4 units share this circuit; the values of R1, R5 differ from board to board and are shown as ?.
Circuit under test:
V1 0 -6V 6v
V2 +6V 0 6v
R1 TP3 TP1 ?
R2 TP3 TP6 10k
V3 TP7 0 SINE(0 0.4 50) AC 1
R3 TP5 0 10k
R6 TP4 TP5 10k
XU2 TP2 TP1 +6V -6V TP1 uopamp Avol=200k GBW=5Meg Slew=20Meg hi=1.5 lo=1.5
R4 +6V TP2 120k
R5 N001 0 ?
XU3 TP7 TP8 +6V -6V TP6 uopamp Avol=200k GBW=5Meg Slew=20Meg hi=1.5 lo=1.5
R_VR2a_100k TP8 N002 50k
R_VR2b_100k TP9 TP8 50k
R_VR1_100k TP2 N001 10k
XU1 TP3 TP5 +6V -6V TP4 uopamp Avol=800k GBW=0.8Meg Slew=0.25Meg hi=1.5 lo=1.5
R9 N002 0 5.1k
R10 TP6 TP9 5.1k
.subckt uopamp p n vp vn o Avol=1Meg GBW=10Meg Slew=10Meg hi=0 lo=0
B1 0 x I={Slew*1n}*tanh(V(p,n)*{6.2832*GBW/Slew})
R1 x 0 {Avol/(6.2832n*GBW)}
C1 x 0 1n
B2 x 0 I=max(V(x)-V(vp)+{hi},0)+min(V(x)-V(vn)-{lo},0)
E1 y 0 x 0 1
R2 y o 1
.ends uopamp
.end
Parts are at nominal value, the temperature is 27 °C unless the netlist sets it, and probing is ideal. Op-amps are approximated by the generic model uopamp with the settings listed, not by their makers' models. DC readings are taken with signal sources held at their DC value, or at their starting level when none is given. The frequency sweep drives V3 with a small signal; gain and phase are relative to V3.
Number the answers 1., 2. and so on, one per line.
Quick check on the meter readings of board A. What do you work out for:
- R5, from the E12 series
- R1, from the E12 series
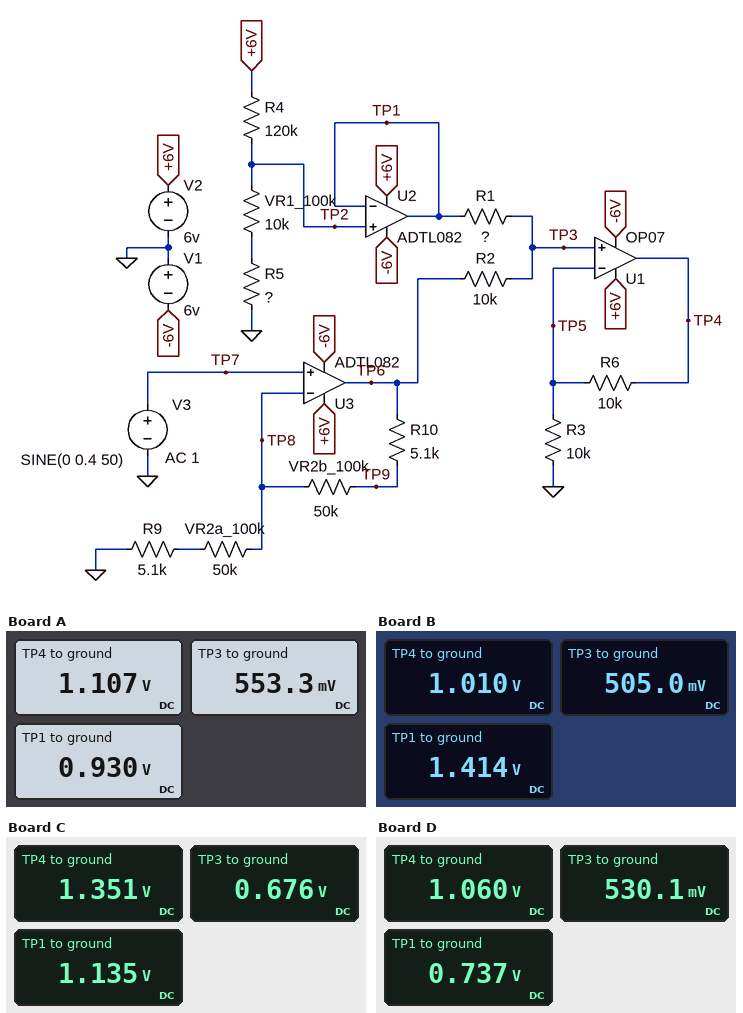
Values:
1. 12 kΩ
2. 6.8 kΩ
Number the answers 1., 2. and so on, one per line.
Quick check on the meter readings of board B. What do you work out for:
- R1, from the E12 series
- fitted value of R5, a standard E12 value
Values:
1. 18 kΩ
2. 27 kΩ
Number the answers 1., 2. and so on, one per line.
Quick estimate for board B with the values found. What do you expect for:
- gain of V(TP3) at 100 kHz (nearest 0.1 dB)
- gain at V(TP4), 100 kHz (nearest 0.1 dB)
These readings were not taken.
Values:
1. 2.2 dB
2. 7.9 dB
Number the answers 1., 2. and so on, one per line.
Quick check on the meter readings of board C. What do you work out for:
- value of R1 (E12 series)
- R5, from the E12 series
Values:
1. 6.8 kΩ
2. 18 kΩ
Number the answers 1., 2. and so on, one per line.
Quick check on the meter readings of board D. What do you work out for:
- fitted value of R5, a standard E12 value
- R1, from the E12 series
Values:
1. 6.8 kΩ
2. 3.9 kΩ
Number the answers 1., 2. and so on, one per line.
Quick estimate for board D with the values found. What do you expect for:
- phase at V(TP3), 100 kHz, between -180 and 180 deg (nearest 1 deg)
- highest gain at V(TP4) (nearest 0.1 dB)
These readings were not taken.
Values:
1. -2 deg
2. 1.0 dB
